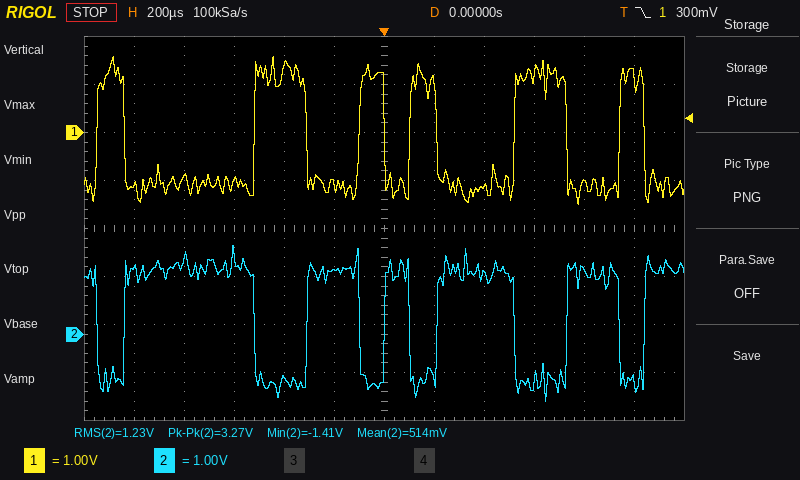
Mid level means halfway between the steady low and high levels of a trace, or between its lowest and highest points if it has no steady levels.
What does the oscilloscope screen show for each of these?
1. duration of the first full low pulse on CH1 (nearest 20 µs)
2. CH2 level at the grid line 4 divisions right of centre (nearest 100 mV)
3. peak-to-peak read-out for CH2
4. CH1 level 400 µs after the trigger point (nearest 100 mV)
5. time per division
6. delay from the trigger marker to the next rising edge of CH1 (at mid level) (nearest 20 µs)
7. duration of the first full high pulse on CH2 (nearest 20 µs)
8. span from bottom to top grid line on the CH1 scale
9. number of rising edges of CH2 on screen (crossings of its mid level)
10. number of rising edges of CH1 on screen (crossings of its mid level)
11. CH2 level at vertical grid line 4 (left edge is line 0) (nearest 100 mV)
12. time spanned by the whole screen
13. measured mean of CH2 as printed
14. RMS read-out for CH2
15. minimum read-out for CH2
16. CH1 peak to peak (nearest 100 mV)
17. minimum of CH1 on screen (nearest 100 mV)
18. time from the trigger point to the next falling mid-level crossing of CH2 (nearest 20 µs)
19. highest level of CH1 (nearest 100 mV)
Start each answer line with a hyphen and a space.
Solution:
- 520 µs
- 1.3 V
- 3.27 V
- -1.1 V
- 200 µs
- 100 µs
- 520 µs
- 8 V
- 6
- 6
- -900 mV
- 2.4 ms
- 514 mV
- 1.23 V
- -1.41 V
- 3.1 V
- -1.5 V
- 100 µs
- 1.6 V
